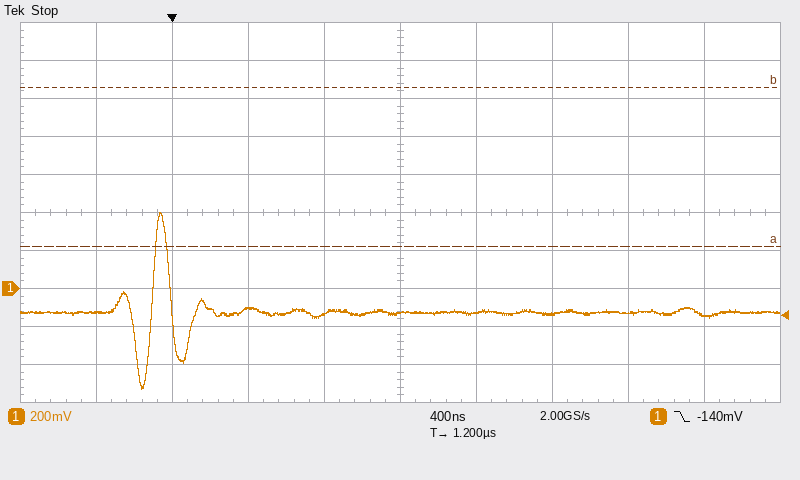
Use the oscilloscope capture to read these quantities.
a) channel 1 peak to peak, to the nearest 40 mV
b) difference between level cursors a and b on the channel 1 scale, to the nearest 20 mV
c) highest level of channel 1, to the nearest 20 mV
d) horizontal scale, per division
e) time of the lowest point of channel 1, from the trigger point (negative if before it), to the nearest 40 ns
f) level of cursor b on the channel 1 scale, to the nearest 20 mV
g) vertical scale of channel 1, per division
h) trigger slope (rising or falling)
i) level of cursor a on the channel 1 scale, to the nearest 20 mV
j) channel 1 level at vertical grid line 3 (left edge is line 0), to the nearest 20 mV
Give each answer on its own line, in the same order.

920 mV
840 mV
400 mV
400 ns
-160 ns
1.06 V
200 mV
falling
220 mV
-100 mV
